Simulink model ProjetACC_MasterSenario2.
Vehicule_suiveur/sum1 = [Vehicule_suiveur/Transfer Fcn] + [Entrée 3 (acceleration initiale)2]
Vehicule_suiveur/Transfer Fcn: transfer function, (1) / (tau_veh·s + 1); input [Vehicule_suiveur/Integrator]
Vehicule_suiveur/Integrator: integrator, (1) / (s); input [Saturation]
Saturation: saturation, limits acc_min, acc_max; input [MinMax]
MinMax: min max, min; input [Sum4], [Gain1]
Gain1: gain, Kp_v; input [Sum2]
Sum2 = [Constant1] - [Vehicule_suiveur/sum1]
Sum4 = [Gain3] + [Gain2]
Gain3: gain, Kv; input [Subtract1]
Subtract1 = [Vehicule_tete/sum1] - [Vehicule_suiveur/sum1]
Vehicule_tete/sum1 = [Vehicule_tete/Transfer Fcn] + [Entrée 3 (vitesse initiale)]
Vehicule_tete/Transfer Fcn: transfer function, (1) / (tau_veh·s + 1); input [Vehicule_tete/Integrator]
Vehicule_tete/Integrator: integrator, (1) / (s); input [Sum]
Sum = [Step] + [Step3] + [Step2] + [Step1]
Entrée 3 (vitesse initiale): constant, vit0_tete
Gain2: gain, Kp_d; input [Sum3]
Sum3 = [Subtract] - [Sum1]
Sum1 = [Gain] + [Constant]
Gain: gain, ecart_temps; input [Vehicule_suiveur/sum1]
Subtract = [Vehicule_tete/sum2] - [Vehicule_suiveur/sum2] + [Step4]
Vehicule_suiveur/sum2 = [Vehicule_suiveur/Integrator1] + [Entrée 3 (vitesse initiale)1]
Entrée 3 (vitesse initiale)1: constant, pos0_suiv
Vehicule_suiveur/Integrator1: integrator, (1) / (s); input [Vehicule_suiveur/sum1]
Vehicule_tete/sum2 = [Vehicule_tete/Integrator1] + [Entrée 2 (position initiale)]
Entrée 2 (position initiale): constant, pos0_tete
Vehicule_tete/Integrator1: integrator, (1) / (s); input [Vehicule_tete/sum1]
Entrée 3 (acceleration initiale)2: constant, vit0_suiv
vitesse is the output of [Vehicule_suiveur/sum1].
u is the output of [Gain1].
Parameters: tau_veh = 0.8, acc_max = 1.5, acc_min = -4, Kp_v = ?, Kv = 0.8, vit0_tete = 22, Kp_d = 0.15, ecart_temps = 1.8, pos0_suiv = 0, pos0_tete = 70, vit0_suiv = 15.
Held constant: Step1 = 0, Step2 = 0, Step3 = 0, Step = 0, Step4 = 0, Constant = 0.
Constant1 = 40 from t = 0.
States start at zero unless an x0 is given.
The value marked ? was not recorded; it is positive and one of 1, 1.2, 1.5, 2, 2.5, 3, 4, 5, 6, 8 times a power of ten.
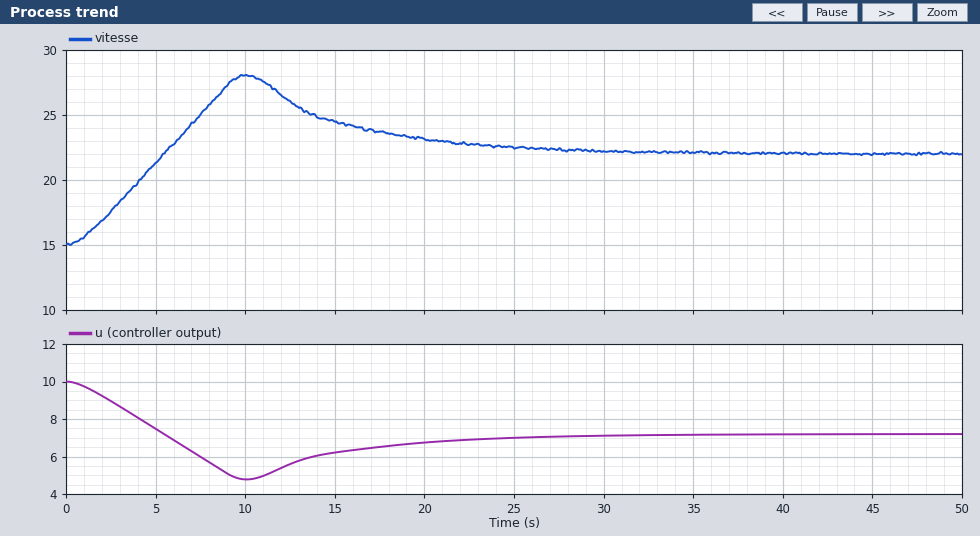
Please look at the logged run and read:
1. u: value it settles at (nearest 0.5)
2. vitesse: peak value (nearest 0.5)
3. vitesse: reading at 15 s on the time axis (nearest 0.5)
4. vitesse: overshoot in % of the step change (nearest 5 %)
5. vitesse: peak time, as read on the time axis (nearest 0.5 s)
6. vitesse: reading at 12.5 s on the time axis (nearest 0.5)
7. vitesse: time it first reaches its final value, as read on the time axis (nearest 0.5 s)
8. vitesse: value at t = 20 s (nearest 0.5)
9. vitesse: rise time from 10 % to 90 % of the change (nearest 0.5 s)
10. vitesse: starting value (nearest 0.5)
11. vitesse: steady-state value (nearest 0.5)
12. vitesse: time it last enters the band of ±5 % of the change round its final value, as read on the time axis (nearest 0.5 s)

7.0
28.0
24.5
85 %
10.0 s
26.0
5.5 s
23.0
4.0 s
15.0
22.0
27.5 s
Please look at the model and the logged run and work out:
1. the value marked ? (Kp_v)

0.4
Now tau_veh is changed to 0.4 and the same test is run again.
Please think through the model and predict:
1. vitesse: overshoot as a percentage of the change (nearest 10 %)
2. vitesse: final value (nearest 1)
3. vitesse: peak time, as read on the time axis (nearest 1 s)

80 %
22
9 s
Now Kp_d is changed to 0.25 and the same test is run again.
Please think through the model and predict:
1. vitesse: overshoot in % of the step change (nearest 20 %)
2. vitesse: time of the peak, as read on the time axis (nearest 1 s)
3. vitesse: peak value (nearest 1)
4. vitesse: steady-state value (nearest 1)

100 %
11 s
29
22
